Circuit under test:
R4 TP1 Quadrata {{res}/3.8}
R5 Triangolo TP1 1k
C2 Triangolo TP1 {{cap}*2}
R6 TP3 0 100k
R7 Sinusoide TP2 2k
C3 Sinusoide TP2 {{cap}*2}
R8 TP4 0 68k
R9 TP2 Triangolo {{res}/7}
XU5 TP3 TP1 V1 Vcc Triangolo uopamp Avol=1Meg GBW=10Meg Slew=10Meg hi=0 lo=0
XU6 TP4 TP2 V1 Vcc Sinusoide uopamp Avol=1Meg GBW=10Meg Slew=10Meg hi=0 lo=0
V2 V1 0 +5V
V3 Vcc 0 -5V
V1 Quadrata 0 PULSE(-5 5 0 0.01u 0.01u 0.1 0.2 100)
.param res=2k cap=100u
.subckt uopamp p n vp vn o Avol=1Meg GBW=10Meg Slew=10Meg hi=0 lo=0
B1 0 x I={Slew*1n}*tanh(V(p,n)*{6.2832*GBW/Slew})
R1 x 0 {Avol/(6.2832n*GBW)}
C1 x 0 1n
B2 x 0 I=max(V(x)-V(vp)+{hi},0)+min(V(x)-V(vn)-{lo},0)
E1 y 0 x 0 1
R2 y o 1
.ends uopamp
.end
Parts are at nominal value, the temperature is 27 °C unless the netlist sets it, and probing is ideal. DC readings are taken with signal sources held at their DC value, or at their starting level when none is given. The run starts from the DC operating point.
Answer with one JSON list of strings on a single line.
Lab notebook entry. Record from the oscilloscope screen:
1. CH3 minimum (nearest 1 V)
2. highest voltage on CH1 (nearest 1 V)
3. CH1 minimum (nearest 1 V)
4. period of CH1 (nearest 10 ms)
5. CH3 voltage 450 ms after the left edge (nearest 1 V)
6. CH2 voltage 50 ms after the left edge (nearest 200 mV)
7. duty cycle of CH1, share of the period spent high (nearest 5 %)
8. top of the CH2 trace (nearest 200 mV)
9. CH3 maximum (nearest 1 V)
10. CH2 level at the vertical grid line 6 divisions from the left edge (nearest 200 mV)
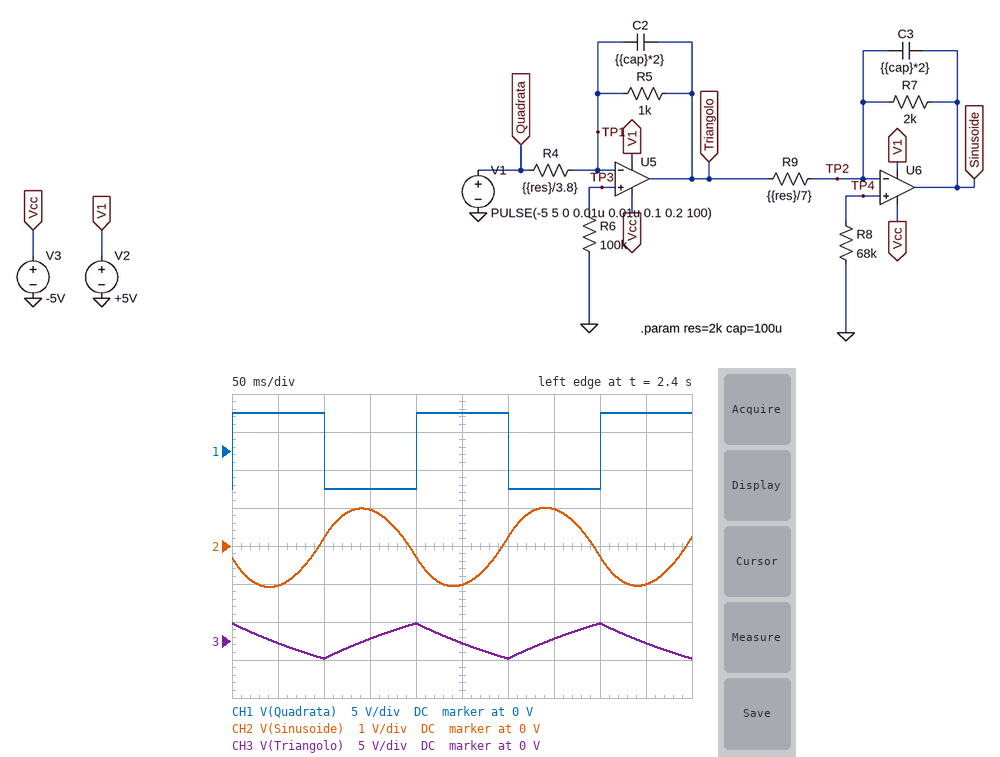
["-2 V", "5 V", "-5 V", "200 ms", "0 V", "-1.0 V", "50 %", "1.0 V", "2 V", "200 mV"]
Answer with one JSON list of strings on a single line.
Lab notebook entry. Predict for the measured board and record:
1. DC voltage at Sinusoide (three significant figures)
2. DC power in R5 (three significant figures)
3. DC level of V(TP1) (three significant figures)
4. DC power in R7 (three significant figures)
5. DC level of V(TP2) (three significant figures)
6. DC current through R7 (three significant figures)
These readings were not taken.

["-5.01 V", "42.9 mW", "-1.55 V", "38.3 mW", "3.75 V", "4.38 mA"]
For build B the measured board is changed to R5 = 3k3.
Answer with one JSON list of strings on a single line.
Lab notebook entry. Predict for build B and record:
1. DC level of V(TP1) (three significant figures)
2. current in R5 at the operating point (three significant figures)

["-3.62 V", "2.61 mA"]
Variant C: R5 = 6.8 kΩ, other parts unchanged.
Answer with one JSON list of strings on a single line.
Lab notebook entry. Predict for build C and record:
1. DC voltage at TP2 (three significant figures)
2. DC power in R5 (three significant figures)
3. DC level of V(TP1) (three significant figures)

["3.75 V", "12.7 mW", "-4.28 V"]
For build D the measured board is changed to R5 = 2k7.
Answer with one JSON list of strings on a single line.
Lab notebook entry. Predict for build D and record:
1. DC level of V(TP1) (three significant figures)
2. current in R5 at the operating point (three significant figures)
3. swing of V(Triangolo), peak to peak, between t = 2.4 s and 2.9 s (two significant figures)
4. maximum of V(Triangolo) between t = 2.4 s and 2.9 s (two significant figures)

["-3.37 V", "3.10 mA", "4.8 V", "2.4 V"]
